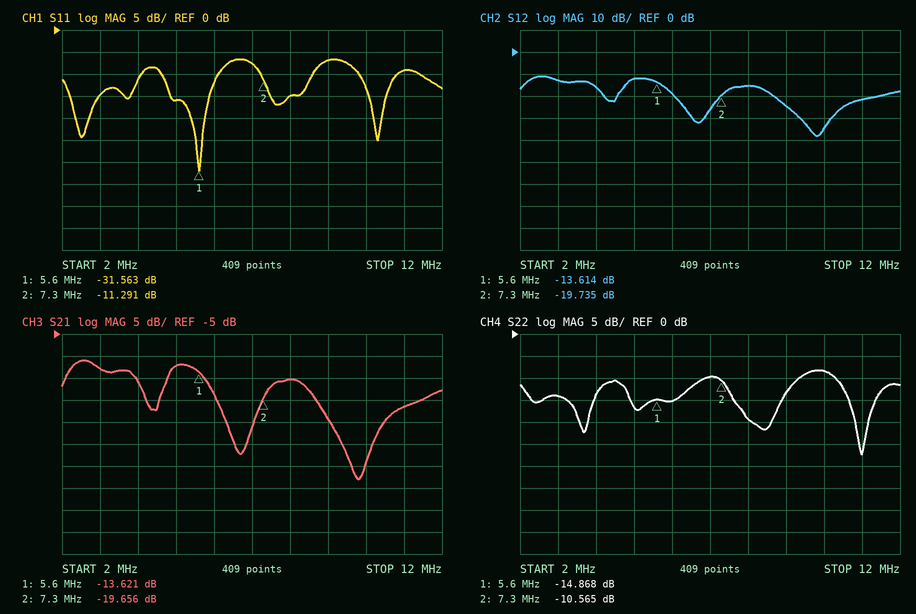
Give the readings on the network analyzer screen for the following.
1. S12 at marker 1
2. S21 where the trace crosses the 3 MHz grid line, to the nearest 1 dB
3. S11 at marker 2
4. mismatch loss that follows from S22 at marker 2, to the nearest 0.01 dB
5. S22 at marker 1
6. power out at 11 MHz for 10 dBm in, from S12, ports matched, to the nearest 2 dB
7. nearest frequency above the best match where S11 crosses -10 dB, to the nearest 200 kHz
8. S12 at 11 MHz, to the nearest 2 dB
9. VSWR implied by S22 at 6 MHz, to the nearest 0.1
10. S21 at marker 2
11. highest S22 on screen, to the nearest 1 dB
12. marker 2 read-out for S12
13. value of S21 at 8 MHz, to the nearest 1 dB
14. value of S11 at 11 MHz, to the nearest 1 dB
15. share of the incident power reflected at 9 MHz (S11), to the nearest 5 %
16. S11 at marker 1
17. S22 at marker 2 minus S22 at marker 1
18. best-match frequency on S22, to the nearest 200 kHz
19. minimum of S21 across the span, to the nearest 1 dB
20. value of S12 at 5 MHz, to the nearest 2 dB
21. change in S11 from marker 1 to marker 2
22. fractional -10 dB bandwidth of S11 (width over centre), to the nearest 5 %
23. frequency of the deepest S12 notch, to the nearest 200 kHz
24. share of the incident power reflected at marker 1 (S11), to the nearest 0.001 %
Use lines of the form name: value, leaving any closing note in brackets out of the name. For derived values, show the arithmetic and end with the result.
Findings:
S12 at marker 1: -13.614 dB
S21 where the trace crosses the 3 MHz grid line, to the nearest 1 dB: -13 dB
S11 at marker 2: -11.291 dB
mismatch loss that follows from S22 at marker 2, to the nearest 0.01 dB: −10 log10(1 − 10^(-10.565/10)) ≈ 0.40 dB
S22 at marker 1: -14.868 dB
power out at 11 MHz for 10 dBm in, from S12, ports matched, to the nearest 2 dB: 10 dBm + (-22 dB) = -12 dBm
nearest frequency above the best match where S11 crosses -10 dB, to the nearest 200 kHz: 6.2 MHz
S12 at 11 MHz, to the nearest 2 dB: -22 dB
VSWR implied by S22 at 6 MHz, to the nearest 0.1: |Γ| = 10^(-15/20) = 0.1778; VSWR = (1 + 0.1778)/(1 − 0.1778) ≈ 1.4
S21 at marker 2: -19.656 dB
highest S22 on screen, to the nearest 1 dB: -8 dB
marker 2 read-out for S12: -19.735 dB
value of S21 at 8 MHz, to the nearest 1 dB: -15 dB
value of S11 at 11 MHz, to the nearest 1 dB: -9 dB
share of the incident power reflected at 9 MHz (S11), to the nearest 5 %: 10^(-7/10) ≈ 20 %
S11 at marker 1: -31.563 dB
S22 at marker 2 minus S22 at marker 1: -10.565 − (-14.868) = 4.303 dB
best-match frequency on S22, to the nearest 200 kHz: 11.0 MHz
minimum of S21 across the span, to the nearest 1 dB: -38 dB
value of S12 at 5 MHz, to the nearest 2 dB: -12 dB
change in S11 from marker 1 to marker 2: -11.291 − (-31.563) = 20.272 dB
fractional -10 dB bandwidth of S11 (width over centre), to the nearest 5 %: 1.6 MHz / 5.4 MHz ≈ 30 %
frequency of the deepest S12 notch, to the nearest 200 kHz: 9.8 MHz
share of the incident power reflected at marker 1 (S11), to the nearest 0.001 %: 10^(-31.563/10) ≈ 0.070 %
